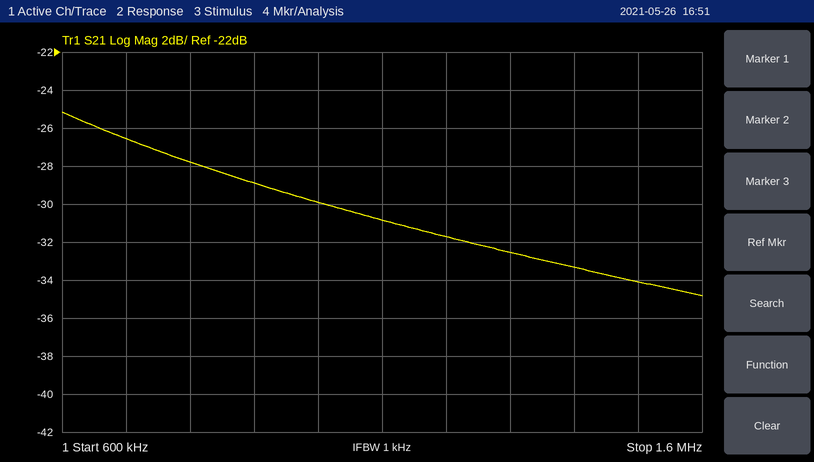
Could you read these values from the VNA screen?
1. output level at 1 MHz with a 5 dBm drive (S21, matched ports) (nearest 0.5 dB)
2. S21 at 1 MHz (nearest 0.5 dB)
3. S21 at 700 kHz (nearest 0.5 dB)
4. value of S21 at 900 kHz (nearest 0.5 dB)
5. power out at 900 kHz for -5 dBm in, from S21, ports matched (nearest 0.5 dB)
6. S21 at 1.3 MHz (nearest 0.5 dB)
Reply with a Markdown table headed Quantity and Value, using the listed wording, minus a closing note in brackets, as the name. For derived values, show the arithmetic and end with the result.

| Quantity | Value |
|---|---|
| output level at 1 MHz with a 5 dBm drive (S21, matched ports) | 5 dBm + (-30.0 dB) = -25.0 dBm |
| S21 at 1 MHz | -30.0 dB |
| S21 at 700 kHz | -26.5 dB |
| value of S21 at 900 kHz | -29.0 dB |
| power out at 900 kHz for -5 dBm in, from S21, ports matched | -5 dBm + (-29.0 dB) = -34.0 dBm |
| S21 at 1.3 MHz | -32.5 dB |
